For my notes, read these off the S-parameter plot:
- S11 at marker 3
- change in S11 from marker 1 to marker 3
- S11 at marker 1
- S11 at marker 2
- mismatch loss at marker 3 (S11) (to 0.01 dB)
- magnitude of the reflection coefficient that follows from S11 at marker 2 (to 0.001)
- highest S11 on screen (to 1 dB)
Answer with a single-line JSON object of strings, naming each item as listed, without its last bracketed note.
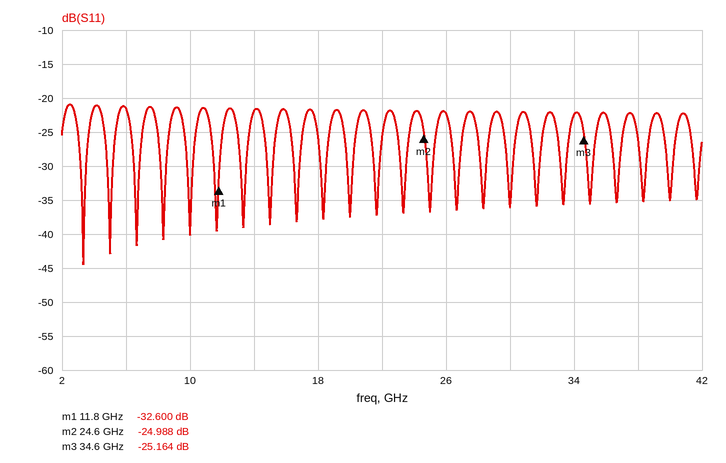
{"S11 at marker 3": "-25.164 dB", "change in S11 from marker 1 to marker 3": "7.436 dB", "S11 at marker 1": "-32.600 dB", "S11 at marker 2": "-24.988 dB", "mismatch loss at marker 3 (S11)": "0.01 dB", "magnitude of the reflection coefficient that follows from S11 at marker 2": "0.056", "highest S11 on screen": "-21 dB"}
